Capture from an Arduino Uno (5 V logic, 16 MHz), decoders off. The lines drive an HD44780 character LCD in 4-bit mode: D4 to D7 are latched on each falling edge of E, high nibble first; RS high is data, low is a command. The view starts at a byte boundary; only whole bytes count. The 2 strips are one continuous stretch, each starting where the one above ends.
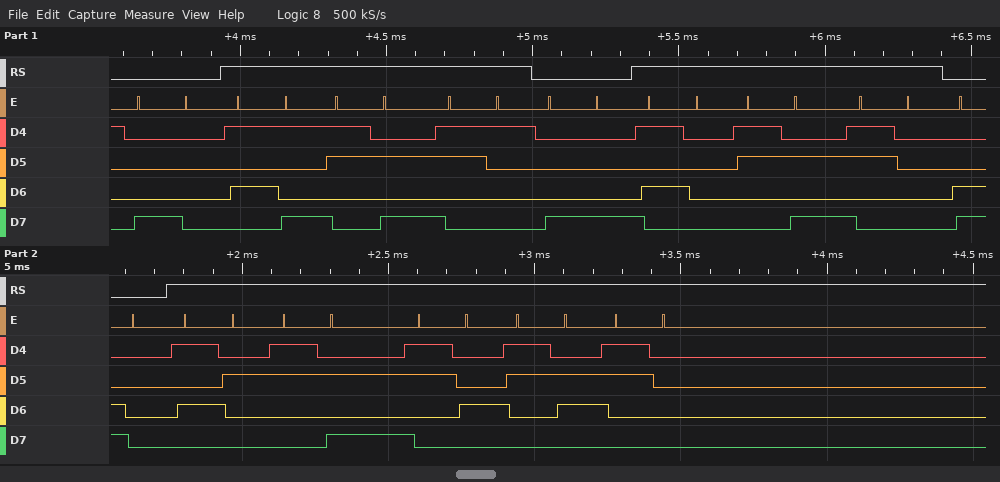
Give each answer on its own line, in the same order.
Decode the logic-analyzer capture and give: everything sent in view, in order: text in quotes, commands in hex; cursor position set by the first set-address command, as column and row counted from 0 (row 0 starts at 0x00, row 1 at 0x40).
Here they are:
0x80 "Y:1" 0x88 "P:0" 0xC0 "R:460"
column 0, row 0
